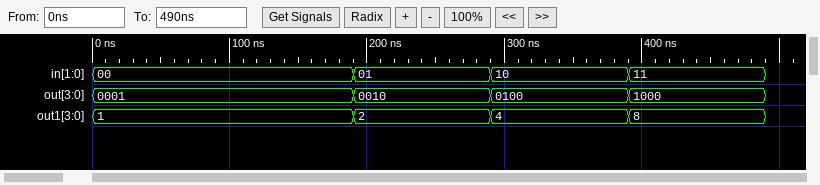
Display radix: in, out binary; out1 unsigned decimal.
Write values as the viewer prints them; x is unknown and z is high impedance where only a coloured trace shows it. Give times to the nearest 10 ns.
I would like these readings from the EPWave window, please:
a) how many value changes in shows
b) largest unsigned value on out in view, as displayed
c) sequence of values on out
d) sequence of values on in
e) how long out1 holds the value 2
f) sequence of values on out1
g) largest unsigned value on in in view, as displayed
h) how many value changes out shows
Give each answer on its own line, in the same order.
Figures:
3
1000
0001, 0010, 0100, 1000
00, 01, 10, 11
100 ns
1, 2, 4, 8
11
3
